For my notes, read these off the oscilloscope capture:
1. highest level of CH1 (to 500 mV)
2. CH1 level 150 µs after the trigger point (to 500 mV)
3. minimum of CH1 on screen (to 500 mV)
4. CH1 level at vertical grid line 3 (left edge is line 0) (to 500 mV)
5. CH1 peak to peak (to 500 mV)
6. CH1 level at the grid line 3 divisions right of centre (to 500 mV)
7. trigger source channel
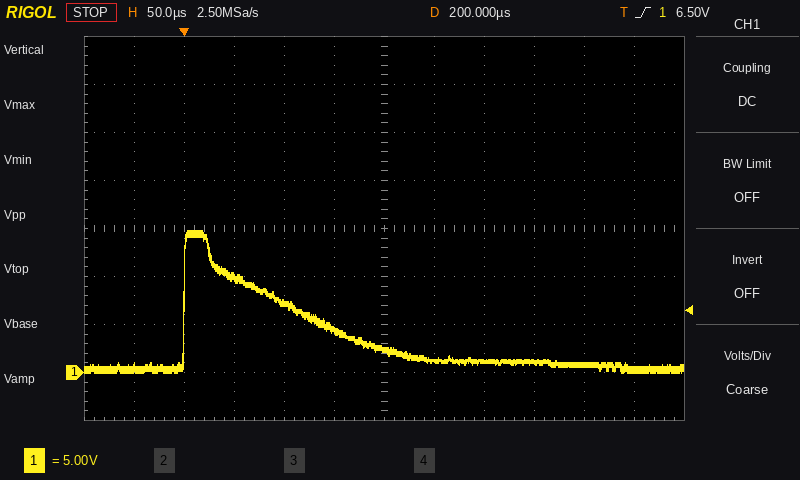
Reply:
15.0 V
4.5 V
0.0 V
10.0 V
15.0 V
1.0 V
CH1
